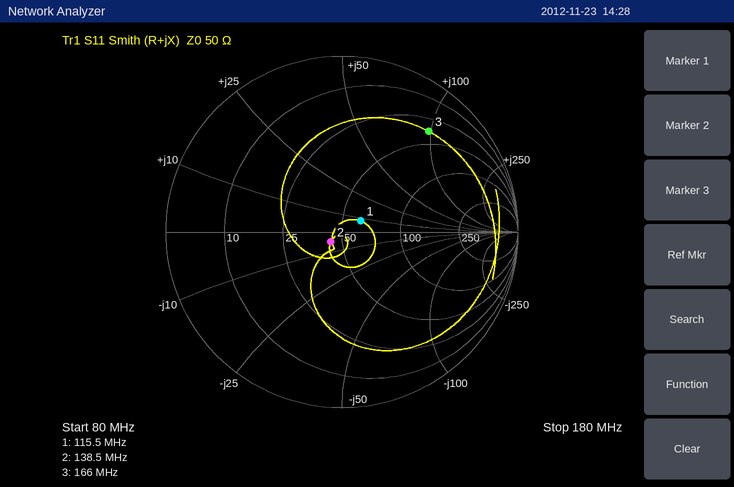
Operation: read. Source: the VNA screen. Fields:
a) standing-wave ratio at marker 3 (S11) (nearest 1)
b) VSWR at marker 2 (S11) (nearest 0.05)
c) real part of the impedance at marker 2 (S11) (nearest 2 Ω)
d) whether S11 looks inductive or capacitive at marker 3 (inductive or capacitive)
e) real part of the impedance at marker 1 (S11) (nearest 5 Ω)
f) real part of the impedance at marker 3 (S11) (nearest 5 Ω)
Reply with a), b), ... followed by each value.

a) 7
b) 1.20
c) 44 Ω
d) inductive
e) 60 Ω
f) 35 Ω
